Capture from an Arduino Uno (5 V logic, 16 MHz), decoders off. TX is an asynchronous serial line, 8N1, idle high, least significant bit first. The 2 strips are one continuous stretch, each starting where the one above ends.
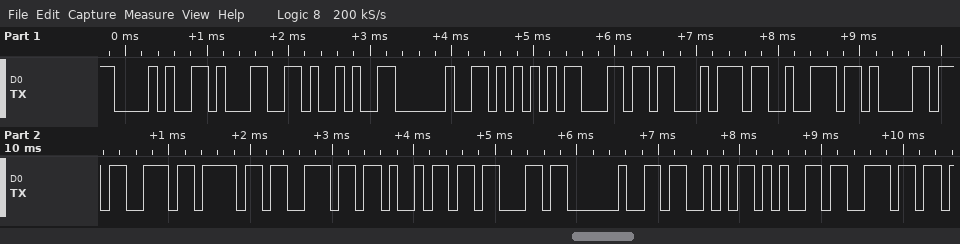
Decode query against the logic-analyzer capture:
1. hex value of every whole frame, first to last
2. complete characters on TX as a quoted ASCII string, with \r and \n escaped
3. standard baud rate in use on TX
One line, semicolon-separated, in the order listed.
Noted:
28 31 29 20 55 6C 74 72 61 73 6F 6E 69 63 20 53 65 6E; "(1) Ultrasonic Sen"; 9600 baud
